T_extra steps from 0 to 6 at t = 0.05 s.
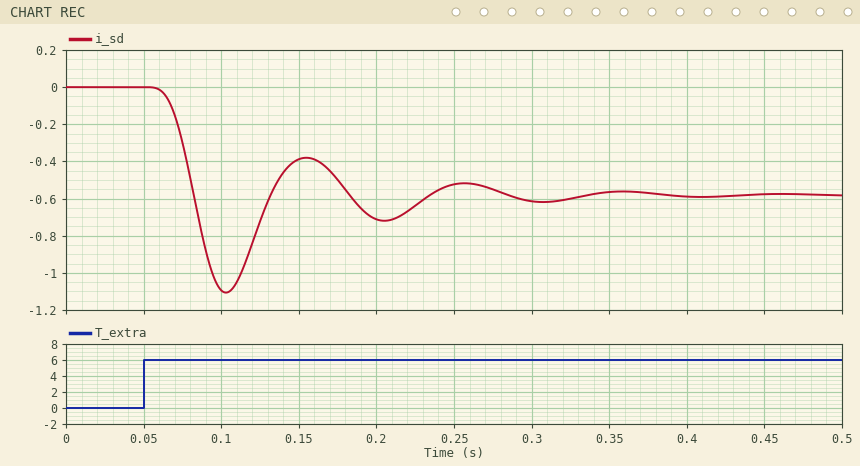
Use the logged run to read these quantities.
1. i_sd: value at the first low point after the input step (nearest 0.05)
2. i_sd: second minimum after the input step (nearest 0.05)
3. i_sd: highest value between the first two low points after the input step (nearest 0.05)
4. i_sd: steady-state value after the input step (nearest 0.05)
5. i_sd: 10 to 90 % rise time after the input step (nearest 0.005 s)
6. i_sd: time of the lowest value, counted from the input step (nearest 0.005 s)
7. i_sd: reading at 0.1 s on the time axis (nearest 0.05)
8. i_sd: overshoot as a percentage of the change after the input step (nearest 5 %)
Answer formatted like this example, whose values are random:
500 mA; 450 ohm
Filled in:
-1.10; -0.70; -0.40; -0.60; 0.015 s; 0.055 s; -1.10; 90 %
